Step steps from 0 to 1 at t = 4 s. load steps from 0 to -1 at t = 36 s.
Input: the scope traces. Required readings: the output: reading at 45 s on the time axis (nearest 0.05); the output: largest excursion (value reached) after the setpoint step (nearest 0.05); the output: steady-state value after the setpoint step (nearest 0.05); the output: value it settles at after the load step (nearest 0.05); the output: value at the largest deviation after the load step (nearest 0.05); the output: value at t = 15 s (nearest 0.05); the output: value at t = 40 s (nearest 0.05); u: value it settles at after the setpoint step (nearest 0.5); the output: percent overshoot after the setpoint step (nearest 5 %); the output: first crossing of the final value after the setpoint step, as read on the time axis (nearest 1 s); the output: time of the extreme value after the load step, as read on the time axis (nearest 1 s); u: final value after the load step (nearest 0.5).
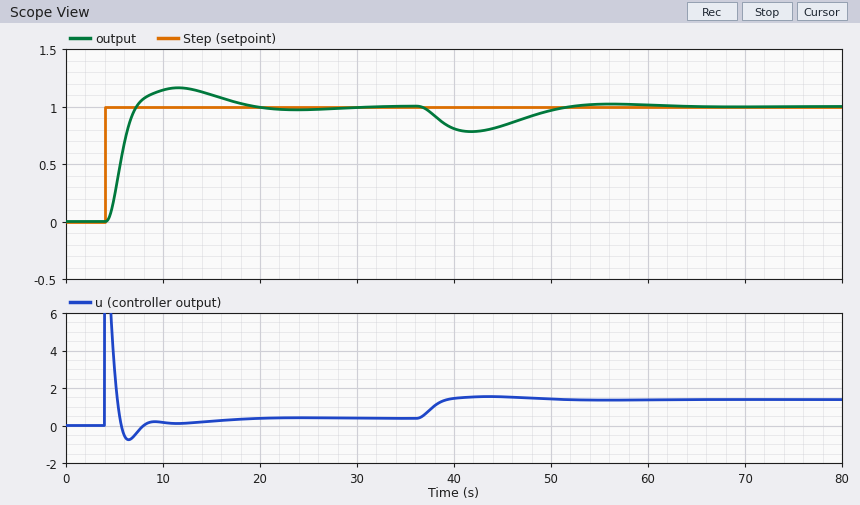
0.85
1.15
1.00
1.00
0.80
1.10
0.80
0.5
15 %
7 s
42 s
1.5
